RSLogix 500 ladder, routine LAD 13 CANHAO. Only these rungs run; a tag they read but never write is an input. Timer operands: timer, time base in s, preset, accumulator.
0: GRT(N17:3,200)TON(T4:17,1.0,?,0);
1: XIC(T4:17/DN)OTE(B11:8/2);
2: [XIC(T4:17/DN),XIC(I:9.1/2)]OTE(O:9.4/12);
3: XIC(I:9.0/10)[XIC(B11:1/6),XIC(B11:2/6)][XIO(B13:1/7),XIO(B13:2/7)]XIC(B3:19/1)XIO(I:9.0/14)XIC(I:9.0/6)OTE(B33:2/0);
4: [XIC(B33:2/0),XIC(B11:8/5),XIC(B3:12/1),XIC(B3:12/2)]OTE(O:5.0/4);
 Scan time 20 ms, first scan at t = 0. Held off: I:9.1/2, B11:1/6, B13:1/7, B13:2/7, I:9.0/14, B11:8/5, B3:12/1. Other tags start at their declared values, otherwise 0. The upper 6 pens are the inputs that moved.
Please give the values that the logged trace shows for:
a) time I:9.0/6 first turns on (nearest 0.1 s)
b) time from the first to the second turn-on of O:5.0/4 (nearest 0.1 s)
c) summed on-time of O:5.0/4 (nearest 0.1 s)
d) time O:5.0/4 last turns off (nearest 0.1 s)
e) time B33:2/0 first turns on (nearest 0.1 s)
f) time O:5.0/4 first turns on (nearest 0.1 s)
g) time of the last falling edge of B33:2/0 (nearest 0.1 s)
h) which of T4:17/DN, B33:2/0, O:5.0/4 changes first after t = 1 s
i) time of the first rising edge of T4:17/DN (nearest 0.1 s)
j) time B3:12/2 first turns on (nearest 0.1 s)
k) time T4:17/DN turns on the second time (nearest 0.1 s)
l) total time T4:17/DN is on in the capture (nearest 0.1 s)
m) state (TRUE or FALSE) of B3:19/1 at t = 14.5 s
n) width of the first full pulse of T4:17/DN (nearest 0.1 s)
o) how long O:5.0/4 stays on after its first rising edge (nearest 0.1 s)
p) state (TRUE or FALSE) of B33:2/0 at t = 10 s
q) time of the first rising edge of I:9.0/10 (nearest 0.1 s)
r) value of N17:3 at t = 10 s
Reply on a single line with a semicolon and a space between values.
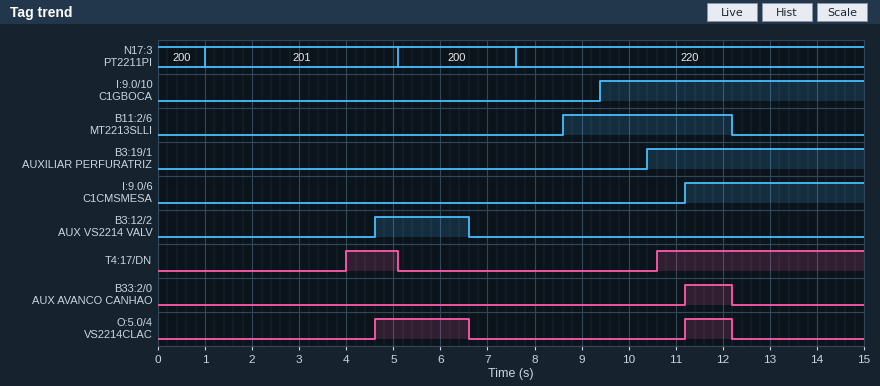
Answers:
11.2 s; 6.6 s; 3.0 s; 12.2 s; 11.2 s; 4.6 s; 12.2 s; T4:17/DN; 4.0 s; 4.6 s; 10.6 s; 5.5 s; TRUE; 1.1 s; 2.0 s; FALSE; 9.4 s; 220
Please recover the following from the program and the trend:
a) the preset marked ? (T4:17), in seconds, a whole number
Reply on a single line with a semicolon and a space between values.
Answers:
3 s
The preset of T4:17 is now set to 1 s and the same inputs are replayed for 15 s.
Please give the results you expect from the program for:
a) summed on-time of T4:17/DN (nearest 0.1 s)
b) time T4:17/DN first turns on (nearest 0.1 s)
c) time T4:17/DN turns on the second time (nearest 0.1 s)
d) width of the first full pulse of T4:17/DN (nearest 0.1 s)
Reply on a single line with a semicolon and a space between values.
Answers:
9.5 s; 2.0 s; 8.6 s; 3.1 s
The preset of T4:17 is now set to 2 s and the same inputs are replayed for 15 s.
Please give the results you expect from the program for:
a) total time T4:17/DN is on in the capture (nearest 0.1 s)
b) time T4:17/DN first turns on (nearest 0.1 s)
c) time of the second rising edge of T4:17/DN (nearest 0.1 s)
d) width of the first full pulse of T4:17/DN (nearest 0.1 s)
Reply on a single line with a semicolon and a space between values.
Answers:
7.5 s; 3.0 s; 9.6 s; 2.1 s
